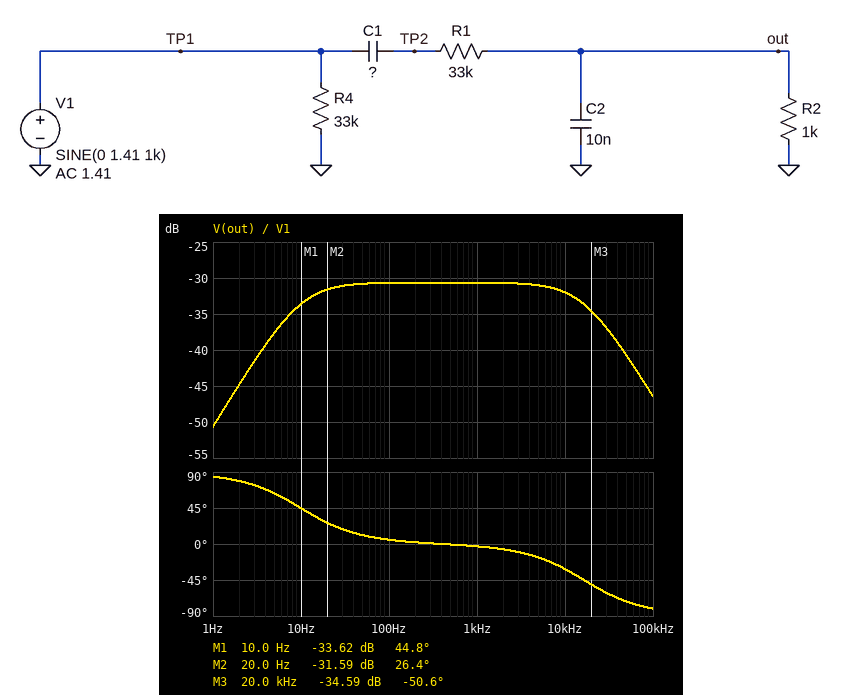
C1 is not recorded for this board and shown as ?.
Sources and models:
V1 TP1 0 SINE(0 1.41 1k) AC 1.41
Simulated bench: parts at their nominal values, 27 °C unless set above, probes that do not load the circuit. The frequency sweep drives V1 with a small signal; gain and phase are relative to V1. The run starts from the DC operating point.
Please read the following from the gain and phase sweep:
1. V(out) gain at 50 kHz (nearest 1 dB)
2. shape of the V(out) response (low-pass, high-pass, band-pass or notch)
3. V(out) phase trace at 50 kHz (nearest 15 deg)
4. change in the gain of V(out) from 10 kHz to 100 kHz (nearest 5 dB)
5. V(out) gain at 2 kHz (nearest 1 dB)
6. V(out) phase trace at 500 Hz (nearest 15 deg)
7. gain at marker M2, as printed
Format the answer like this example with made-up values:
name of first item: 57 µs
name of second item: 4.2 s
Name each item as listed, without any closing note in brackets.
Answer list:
V(out) gain at 50 kHz: -41 dB
shape of the V(out) response: band-pass
V(out) phase trace at 50 kHz: -75 deg
change in the gain of V(out) from 10 kHz to 100 kHz: -15 dB
V(out) gain at 2 kHz: -31 dB
V(out) phase trace at 500 Hz: 0 deg
gain at marker M2, as printed: -31.59 dB
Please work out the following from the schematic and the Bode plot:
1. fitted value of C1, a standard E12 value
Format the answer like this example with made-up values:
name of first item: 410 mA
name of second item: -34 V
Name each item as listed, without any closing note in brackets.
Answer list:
fitted value of C1, a standard E12 value: 470 nF
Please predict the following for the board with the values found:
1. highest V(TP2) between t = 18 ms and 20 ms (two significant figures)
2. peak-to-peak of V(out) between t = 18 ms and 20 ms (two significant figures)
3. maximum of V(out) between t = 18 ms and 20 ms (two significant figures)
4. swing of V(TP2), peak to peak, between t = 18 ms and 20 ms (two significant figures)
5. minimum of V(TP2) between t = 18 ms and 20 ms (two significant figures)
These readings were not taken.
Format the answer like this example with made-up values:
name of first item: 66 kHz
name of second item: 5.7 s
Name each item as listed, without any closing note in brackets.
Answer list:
highest V(TP2) between t = 18 ms and 20 ms: 1.4 V
peak-to-peak of V(out) between t = 18 ms and 20 ms: 83 mV
maximum of V(out) between t = 18 ms and 20 ms: 41 mV
swing of V(TP2), peak to peak, between t = 18 ms and 20 ms: 2.8 V
minimum of V(TP2) between t = 18 ms and 20 ms: -1.4 V
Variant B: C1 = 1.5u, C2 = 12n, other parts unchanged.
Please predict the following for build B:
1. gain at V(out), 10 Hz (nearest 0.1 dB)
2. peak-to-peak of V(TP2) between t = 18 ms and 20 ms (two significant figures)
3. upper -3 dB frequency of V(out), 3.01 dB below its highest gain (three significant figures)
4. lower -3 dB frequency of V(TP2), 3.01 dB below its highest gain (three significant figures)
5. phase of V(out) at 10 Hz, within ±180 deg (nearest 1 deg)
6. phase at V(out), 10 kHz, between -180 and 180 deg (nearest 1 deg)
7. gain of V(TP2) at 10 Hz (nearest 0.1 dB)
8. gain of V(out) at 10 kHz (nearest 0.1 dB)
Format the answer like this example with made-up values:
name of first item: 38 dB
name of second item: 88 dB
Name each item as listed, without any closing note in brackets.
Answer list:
gain at V(out), 10 Hz: -31.0 dB
peak-to-peak of V(TP2) between t = 18 ms and 20 ms: 2.8 V
upper -3 dB frequency of V(out), 3.01 dB below its highest gain: 13.7 kHz
lower -3 dB frequency of V(TP2), 3.01 dB below its highest gain: 3.12 Hz
phase of V(out) at 10 Hz, within ±180 deg: 17 deg
phase at V(out), 10 kHz, between -180 and 180 deg: -36 deg
gain of V(TP2) at 10 Hz: -0.4 dB
gain of V(out) at 10 kHz: -32.5 dB
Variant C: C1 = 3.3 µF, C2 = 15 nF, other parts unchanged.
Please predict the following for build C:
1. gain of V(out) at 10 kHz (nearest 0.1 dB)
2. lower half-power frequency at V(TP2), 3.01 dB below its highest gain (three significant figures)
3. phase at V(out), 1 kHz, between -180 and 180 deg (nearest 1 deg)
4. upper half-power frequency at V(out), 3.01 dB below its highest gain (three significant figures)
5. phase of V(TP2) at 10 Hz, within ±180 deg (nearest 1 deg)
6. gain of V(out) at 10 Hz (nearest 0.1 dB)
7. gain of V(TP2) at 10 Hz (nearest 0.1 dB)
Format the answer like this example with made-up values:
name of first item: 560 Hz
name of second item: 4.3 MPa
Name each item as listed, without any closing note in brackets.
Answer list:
gain of V(out) at 10 kHz: -33.3 dB
lower half-power frequency at V(TP2), 3.01 dB below its highest gain: 1.42 Hz
phase at V(out), 1 kHz, between -180 and 180 deg: -5 deg
upper half-power frequency at V(out), 3.01 dB below its highest gain: 10.9 kHz
phase of V(TP2) at 10 Hz, within ±180 deg: 8 deg
gain of V(out) at 10 Hz: -30.7 dB
gain of V(TP2) at 10 Hz: -0.1 dB
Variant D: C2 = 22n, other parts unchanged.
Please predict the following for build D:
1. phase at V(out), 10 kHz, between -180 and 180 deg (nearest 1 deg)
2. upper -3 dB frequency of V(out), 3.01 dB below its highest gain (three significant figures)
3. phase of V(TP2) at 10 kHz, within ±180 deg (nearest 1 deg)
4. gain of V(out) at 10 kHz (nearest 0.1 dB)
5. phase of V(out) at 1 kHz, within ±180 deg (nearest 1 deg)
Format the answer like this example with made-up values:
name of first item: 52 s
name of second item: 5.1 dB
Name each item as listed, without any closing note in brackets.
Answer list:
phase at V(out), 10 kHz, between -180 and 180 deg: -53 deg
upper -3 dB frequency of V(out), 3.01 dB below its highest gain: 7.47 kHz
phase of V(TP2) at 10 kHz, within ±180 deg: 0 deg
gain of V(out) at 10 kHz: -35.1 dB
phase of V(out) at 1 kHz, within ±180 deg: -7 deg
